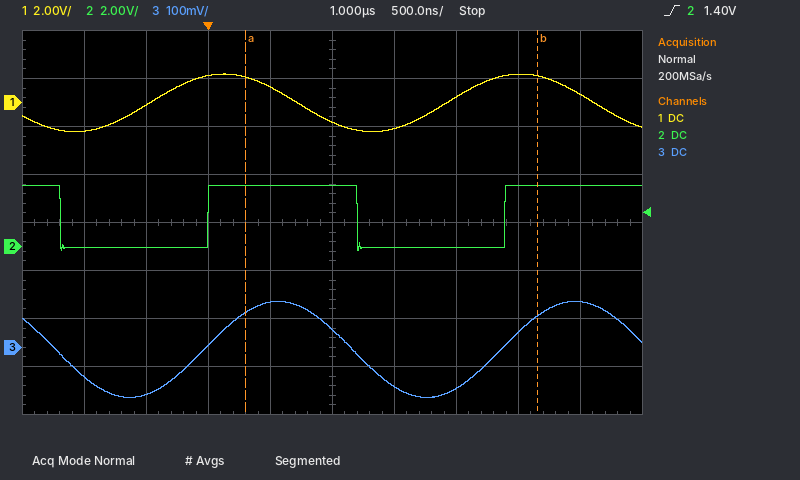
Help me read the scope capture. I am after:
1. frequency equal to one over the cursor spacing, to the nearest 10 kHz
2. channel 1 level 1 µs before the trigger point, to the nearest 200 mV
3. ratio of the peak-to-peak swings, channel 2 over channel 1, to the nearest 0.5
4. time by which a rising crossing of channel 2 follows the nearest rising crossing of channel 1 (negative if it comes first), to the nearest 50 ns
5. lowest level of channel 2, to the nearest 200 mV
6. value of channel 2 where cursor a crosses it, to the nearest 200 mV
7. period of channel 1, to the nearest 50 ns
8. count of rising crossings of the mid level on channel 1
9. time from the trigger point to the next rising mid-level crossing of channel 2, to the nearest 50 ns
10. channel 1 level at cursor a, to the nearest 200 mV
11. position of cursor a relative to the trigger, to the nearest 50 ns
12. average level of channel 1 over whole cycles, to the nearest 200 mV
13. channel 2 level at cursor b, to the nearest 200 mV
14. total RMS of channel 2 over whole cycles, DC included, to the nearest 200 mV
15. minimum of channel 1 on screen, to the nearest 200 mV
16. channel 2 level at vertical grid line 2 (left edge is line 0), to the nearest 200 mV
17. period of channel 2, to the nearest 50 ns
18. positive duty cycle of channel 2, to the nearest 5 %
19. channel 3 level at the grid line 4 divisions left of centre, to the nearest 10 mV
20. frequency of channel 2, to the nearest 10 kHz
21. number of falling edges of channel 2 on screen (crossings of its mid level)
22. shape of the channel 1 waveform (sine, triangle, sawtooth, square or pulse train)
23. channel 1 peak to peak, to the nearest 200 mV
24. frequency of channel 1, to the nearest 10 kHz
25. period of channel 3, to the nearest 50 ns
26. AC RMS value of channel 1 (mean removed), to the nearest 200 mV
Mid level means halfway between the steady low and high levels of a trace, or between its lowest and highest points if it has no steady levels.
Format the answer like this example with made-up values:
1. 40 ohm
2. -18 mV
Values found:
1. 430 kHz
2. -1.2 V
3. 1.0
4. +450 ns
5. -200 mV
6. 2.6 V
7. 2.40 µs
8. 2
9. 2.40 µs
10. 1.0 V
11. +300 ns
12. 0.0 V
13. 2.6 V
14. 1.8 V
15. -1.2 V
16. 0.0 V
17. 2.40 µs
18. 50 %
19. -60 mV
20. 420 kHz
21. 2
22. sine
23. 2.4 V
24. 420 kHz
25. 2.40 µs
26. 800 mV
